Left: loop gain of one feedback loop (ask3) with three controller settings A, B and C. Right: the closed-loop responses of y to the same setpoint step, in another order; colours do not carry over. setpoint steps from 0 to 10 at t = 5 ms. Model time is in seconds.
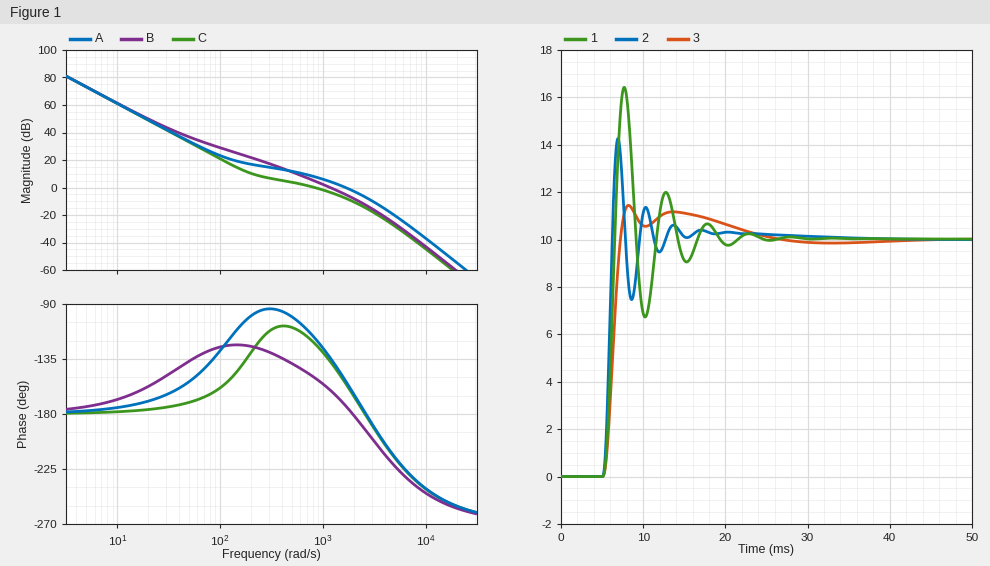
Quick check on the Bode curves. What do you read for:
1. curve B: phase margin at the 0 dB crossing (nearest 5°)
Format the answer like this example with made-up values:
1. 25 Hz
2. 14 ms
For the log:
1. 20°
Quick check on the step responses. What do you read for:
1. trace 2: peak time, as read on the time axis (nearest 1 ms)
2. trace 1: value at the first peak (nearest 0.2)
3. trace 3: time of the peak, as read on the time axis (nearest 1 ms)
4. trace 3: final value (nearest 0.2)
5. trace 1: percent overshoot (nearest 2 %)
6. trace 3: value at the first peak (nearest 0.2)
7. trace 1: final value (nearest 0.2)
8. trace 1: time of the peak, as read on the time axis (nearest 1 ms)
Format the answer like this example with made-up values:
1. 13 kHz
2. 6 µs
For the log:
1. 7 ms
2. 16.4
3. 8 ms
4. 10.0
5. 64 %
6. 11.4
7. 10.0
8. 8 ms
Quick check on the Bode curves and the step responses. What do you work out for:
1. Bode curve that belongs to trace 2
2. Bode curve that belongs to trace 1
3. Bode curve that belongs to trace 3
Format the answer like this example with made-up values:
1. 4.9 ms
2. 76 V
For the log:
1. A
2. B
3. C
